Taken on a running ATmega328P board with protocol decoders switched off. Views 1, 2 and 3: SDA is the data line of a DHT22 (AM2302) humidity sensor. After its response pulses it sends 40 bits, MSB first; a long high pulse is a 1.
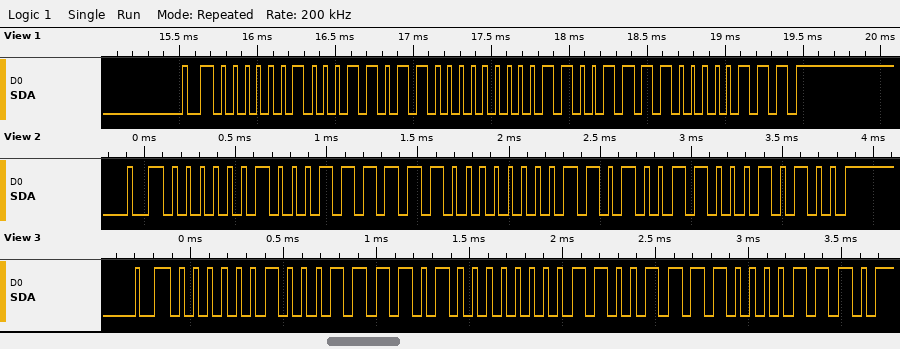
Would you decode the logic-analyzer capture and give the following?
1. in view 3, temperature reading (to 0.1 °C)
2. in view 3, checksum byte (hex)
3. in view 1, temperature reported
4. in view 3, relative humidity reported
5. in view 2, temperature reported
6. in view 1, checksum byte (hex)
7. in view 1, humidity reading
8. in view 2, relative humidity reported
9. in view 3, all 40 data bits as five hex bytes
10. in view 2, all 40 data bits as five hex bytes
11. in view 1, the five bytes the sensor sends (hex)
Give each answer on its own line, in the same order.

20.7 °C
0x0E
20.7 °C
57.3 %
21.1 °C
0x07
56.6 %
57.5 %
02 3D 00 CF 0E
02 3F 00 D3 14
02 36 00 CF 07
